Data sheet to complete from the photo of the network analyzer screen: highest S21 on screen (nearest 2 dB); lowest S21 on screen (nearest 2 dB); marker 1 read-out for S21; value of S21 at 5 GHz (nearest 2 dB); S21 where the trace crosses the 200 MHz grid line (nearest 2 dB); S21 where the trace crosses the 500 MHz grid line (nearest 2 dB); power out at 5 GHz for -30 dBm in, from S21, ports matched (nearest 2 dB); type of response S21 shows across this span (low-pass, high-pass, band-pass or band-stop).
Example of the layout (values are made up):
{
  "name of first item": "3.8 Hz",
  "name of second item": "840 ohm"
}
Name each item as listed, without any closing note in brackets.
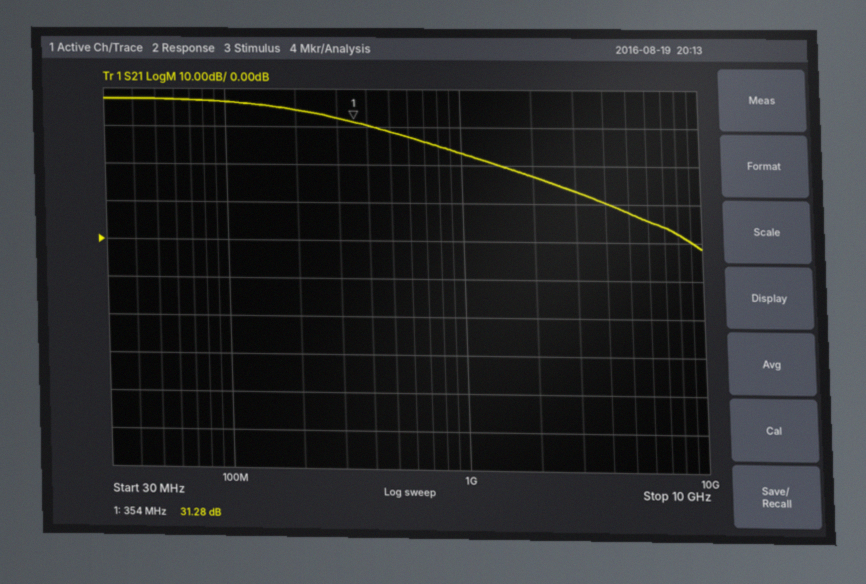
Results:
{
  "highest S21 on screen": "38 dB",
  "lowest S21 on screen": "-2 dB",
  "marker 1 read-out for S21": "31.28 dB",
  "value of S21 at 5 GHz": "8 dB",
  "S21 where the trace crosses the 200 MHz grid line": "34 dB",
  "S21 where the trace crosses the 500 MHz grid line": "28 dB",
  "power out at 5 GHz for -30 dBm in, from S21, ports matched": "-22 dBm",
  "type of response S21 shows across this span": "low-pass"
}
